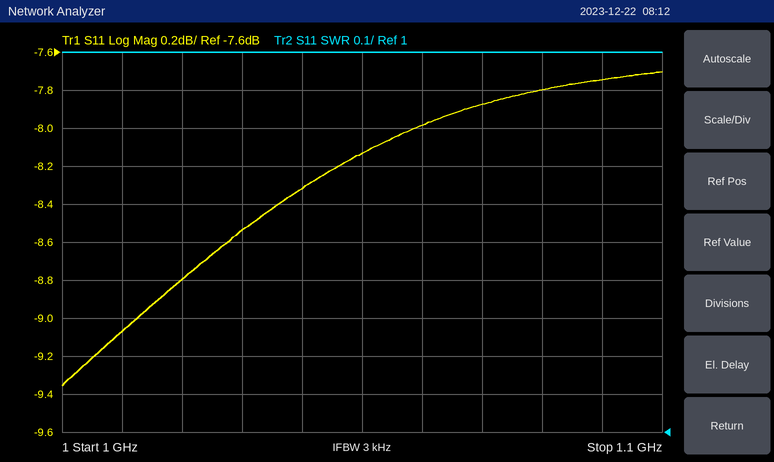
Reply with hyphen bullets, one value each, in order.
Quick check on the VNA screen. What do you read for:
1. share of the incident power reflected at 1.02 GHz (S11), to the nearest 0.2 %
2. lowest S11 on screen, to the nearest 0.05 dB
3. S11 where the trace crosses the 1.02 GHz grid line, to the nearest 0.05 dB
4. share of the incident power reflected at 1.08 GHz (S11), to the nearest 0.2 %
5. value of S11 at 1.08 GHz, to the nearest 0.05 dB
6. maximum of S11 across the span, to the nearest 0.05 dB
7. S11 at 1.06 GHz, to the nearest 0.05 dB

- 13.2 %
- -9.35 dB
- -8.80 dB
- 16.6 %
- -7.80 dB
- -7.70 dB
- -8.00 dB
